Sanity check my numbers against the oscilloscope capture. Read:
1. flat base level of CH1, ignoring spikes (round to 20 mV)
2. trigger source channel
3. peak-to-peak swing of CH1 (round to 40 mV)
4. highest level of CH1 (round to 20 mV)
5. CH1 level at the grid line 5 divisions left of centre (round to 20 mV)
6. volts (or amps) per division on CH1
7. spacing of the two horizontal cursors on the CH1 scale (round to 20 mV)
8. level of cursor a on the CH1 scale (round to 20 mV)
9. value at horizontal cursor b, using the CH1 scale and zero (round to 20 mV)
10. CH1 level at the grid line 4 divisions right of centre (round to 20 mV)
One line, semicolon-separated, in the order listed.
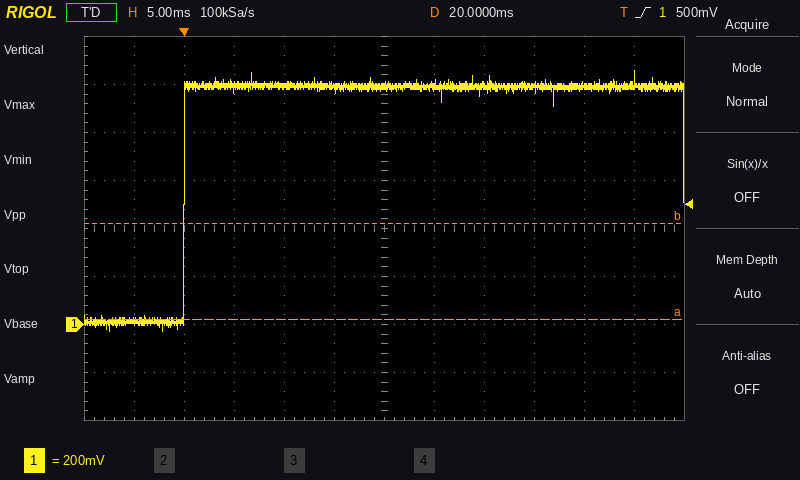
20 mV; CH1; 1.08 V; 1.06 V; 20 mV; 200 mV; 400 mV; 20 mV; 420 mV; 1.00 V
